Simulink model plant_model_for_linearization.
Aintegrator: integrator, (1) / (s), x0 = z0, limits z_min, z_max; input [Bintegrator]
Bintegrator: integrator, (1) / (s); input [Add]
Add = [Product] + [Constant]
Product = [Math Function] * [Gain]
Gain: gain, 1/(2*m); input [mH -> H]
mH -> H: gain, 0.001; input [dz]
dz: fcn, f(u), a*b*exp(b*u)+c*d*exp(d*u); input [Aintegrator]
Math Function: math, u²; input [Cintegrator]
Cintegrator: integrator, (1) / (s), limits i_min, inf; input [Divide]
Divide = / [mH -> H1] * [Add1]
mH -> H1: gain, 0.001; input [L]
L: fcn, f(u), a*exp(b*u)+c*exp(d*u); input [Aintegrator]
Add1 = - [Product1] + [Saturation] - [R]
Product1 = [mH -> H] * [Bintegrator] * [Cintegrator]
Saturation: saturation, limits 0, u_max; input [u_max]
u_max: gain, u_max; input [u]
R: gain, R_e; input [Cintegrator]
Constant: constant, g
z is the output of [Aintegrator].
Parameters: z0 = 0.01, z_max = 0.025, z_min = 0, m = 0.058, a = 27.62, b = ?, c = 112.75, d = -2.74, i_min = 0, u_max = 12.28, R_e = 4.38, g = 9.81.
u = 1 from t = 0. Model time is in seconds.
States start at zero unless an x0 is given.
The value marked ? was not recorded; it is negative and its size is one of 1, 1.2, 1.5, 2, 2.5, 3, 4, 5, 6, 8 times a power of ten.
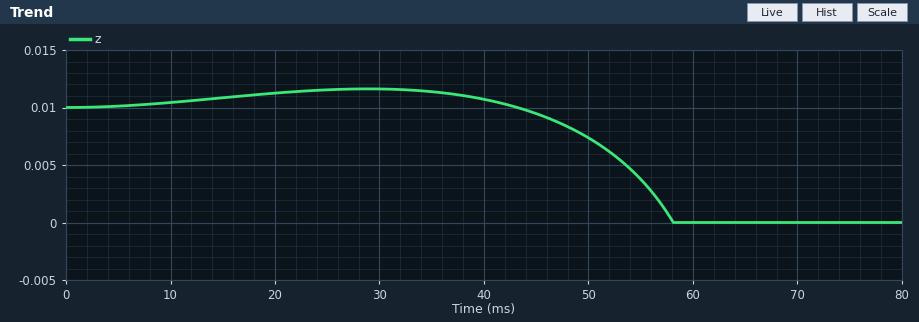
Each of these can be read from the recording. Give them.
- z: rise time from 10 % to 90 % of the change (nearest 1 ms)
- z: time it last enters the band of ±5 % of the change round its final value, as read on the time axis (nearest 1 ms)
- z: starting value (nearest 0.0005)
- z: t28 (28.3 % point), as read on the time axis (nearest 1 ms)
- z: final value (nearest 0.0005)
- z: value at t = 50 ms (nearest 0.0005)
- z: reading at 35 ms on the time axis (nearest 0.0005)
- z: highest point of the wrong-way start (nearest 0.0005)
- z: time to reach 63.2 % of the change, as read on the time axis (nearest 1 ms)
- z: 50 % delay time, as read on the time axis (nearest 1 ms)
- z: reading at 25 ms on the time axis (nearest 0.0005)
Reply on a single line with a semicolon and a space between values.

11 ms; 58 ms; 0.0100; 50 ms; 0.0000; 0.0075; 0.0115; 0.0115; 55 ms; 54 ms; 0.0115
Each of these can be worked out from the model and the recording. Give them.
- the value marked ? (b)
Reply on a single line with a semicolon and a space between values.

-250
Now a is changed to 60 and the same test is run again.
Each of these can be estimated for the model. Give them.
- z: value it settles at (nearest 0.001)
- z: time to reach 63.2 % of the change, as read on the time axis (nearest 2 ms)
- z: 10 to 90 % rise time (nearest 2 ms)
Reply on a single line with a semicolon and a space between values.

0.000; 40 ms; 10 ms
